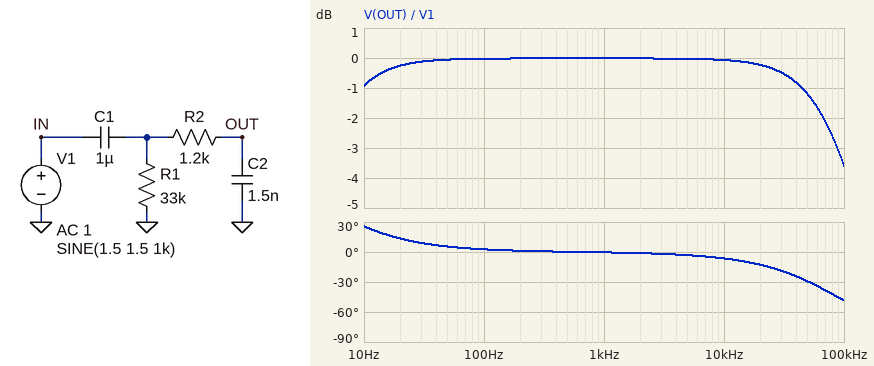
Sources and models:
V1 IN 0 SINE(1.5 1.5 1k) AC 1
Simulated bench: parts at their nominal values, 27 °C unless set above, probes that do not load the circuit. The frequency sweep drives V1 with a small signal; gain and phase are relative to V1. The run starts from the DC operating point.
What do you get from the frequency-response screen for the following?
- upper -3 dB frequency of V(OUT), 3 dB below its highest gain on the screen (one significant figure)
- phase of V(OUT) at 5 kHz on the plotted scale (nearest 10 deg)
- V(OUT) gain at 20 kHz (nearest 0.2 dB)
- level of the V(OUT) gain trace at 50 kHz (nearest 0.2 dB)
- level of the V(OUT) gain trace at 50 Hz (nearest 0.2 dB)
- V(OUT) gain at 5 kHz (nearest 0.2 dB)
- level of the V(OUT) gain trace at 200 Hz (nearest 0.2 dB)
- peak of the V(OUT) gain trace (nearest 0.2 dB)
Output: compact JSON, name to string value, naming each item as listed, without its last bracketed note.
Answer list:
{"upper -3 dB frequency of V(OUT), 3 dB below its highest gain on the screen": "90 kHz", "phase of V(OUT) at 5 kHz on the plotted scale": "0 deg", "V(OUT) gain at 20 kHz": "-0.2 dB", "level of the V(OUT) gain trace at 50 kHz": "-1.2 dB", "level of the V(OUT) gain trace at 50 Hz": "0 dB", "V(OUT) gain at 5 kHz": "0 dB", "level of the V(OUT) gain trace at 200 Hz": "0 dB", "peak of the V(OUT) gain trace": "0 dB"}
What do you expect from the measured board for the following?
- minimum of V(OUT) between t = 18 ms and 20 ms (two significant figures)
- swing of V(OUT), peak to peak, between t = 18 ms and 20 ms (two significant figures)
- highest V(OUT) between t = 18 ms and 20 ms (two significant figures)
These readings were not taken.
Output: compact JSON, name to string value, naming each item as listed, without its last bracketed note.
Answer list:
{"minimum of V(OUT) between t = 18 ms and 20 ms": "-1.5 V", "swing of V(OUT), peak to peak, between t = 18 ms and 20 ms": "3.0 V", "highest V(OUT) between t = 18 ms and 20 ms": "1.5 V"}
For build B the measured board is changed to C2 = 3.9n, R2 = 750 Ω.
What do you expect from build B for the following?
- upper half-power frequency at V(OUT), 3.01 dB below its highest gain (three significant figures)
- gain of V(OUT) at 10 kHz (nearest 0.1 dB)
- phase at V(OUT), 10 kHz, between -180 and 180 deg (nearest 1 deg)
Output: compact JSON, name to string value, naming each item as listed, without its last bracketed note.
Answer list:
{"upper half-power frequency at V(OUT), 3.01 dB below its highest gain": "54.6 kHz", "gain of V(OUT) at 10 kHz": "-0.2 dB", "phase at V(OUT), 10 kHz, between -180 and 180 deg": "-10 deg"}
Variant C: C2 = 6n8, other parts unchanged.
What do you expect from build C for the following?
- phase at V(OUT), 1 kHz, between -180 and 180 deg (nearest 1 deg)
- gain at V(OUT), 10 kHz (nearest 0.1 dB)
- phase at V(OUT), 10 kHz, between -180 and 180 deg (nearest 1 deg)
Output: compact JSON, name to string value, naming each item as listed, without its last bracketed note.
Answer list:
{"phase at V(OUT), 1 kHz, between -180 and 180 deg": "-3 deg", "gain at V(OUT), 10 kHz": "-1.1 dB", "phase at V(OUT), 10 kHz, between -180 and 180 deg": "-27 deg"}
